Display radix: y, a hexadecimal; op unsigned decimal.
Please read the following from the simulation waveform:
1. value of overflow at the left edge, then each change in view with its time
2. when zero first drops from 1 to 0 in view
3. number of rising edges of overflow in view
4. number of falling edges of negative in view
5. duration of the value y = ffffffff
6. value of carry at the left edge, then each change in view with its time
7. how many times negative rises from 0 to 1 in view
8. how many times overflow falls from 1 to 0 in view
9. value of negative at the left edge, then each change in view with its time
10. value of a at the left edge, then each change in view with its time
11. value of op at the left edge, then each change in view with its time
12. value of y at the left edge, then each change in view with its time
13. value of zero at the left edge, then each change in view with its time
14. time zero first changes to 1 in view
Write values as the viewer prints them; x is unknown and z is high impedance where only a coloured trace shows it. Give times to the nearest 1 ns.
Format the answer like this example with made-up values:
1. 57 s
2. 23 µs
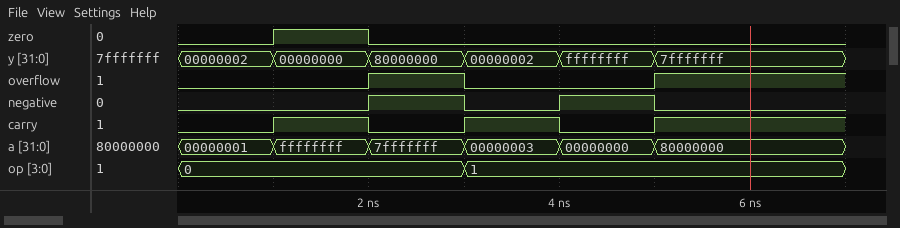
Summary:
1. 0, 1 at 2 ns, 0 at 3 ns, 1 at 5 ns
2. 2 ns
3. 2
4. 2
5. 1 ns
6. 0, 1 at 1 ns, 0 at 2 ns, 1 at 3 ns, 0 at 4 ns, 1 at 5 ns
7. 2
8. 1
9. 0, 1 at 2 ns, 0 at 3 ns, 1 at 4 ns, 0 at 5 ns
10. 00000001, ffffffff at 1 ns, 7fffffff at 2 ns, 00000003 at 3 ns, 00000000 at 4 ns, 80000000 at 5 ns
11. 0, 1 at 3 ns
12. 00000002, 00000000 at 1 ns, 80000000 at 2 ns, 00000002 at 3 ns, ffffffff at 4 ns, 7fffffff at 5 ns
13. 0, 1 at 1 ns, 0 at 2 ns
14. 1 ns
